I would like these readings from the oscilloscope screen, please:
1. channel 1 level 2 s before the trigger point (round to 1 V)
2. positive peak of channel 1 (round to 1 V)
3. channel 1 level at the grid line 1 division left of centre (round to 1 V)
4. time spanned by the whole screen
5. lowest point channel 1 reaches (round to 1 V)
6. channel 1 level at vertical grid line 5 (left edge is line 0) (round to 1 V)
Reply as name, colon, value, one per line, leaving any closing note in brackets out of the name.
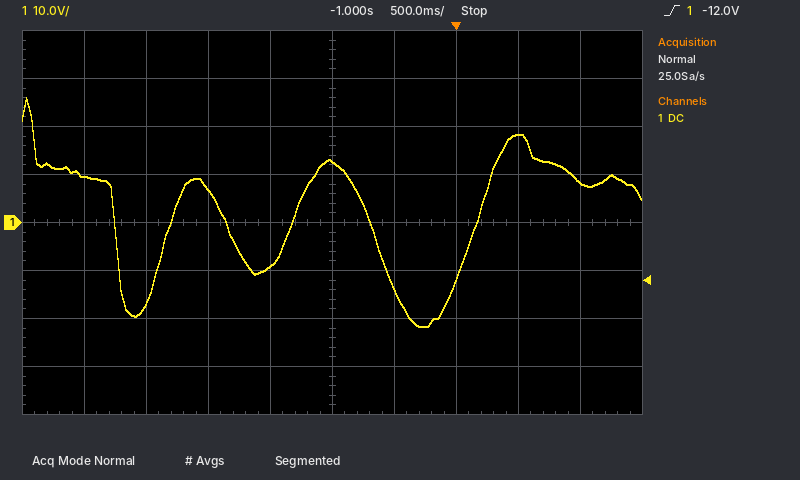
channel 1 level 2 s before the trigger point: 7 V
positive peak of channel 1: 26 V
channel 1 level at the grid line 1 division left of centre: -9 V
time spanned by the whole screen: 5 s
lowest point channel 1 reaches: -22 V
channel 1 level at vertical grid line 5 (left edge is line 0): 13 V
